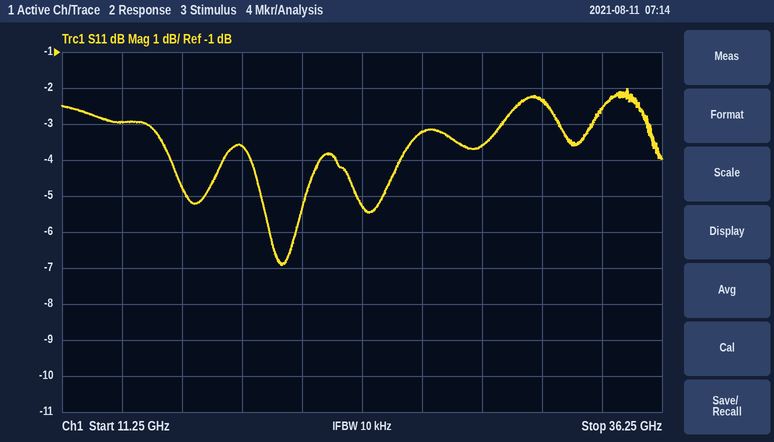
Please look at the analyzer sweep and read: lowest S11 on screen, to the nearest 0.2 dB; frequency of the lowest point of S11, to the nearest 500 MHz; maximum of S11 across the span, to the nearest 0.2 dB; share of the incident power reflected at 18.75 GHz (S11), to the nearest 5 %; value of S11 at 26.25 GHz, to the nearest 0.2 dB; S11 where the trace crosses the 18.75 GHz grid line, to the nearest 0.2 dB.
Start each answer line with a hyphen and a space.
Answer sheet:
- -7.0 dB
- 20.5 GHz
- -2.0 dB
- 45 %
- -3.2 dB
- -3.6 dB
